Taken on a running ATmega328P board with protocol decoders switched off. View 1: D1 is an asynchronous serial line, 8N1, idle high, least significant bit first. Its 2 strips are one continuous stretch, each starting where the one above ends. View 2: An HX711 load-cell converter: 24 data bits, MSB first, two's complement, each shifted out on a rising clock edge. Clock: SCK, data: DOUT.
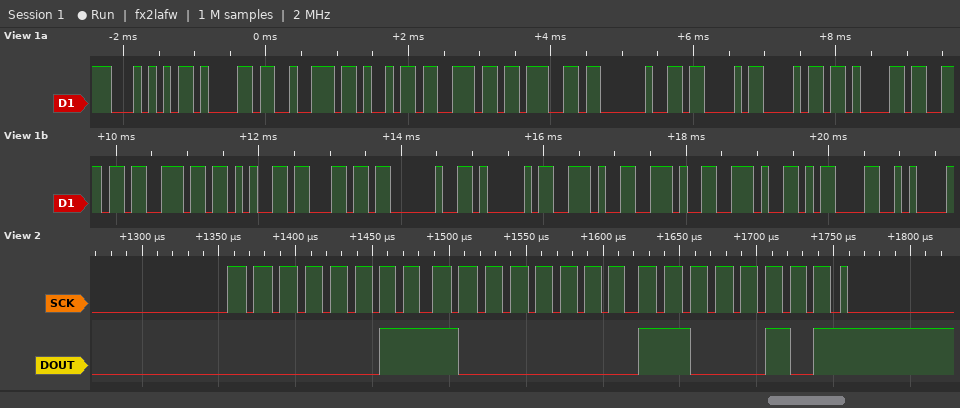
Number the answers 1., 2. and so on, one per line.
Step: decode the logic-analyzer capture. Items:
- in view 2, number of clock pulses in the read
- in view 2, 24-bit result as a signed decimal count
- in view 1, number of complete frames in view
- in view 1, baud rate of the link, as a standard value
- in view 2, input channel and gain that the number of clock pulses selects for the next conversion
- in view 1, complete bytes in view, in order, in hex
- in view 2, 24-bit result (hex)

1. 25
2. 229573
3. 21
4. 9600 baud
5. channel A, gain 128
6. 54 61 72 69 6E 67 20 43 68 61 6E 6E 65 6C 20 41 2E 2E 2E 0D 0A
7. 0x0380C5
